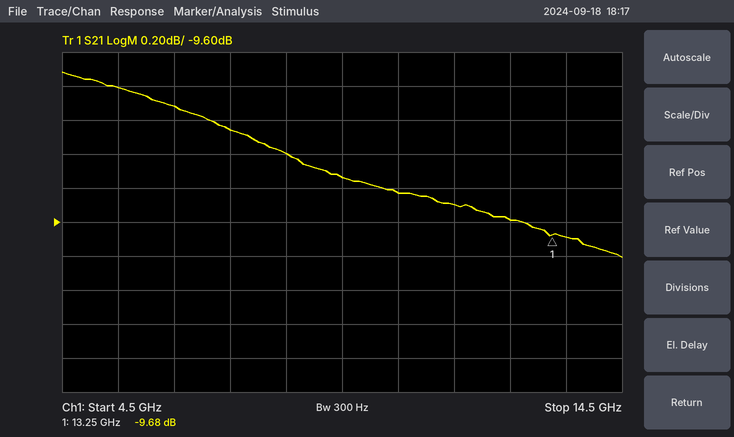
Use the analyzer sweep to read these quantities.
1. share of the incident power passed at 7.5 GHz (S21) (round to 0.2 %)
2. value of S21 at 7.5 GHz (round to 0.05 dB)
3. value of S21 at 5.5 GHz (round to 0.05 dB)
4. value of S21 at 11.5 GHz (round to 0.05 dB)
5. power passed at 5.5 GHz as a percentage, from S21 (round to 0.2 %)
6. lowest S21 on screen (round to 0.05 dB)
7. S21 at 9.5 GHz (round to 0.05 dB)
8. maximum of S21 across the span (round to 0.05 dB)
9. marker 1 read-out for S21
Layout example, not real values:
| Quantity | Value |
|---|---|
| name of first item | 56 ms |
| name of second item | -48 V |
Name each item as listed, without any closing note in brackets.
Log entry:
| Quantity | Value |
|---|---|
| share of the incident power passed at 7.5 GHz (S21) | 12.4 % |
| value of S21 at 7.5 GHz | -9.05 dB |
| value of S21 at 5.5 GHz | -8.80 dB |
| value of S21 at 11.5 GHz | -9.50 dB |
| power passed at 5.5 GHz as a percentage, from S21 | 13.2 % |
| lowest S21 on screen | -9.80 dB |
| S21 at 9.5 GHz | -9.35 dB |
| maximum of S21 across the span | -8.70 dB |
| marker 1 read-out for S21 | -9.68 dB |
